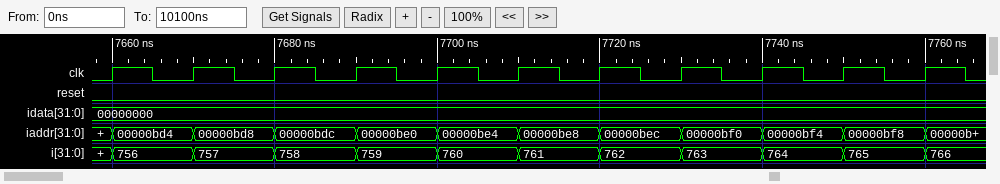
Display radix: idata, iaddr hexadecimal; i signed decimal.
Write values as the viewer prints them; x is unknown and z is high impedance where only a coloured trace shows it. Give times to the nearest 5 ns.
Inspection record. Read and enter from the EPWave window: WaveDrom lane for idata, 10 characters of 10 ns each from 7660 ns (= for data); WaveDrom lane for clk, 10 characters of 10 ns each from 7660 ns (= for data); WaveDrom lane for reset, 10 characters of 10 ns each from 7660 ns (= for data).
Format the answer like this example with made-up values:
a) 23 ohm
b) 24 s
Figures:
a) {name: 'idata', wave: '=.........', data: '00000000'}
b) {name: 'clk', wave: 'p.........'}
c) {name: 'reset', wave: '0.........'}
